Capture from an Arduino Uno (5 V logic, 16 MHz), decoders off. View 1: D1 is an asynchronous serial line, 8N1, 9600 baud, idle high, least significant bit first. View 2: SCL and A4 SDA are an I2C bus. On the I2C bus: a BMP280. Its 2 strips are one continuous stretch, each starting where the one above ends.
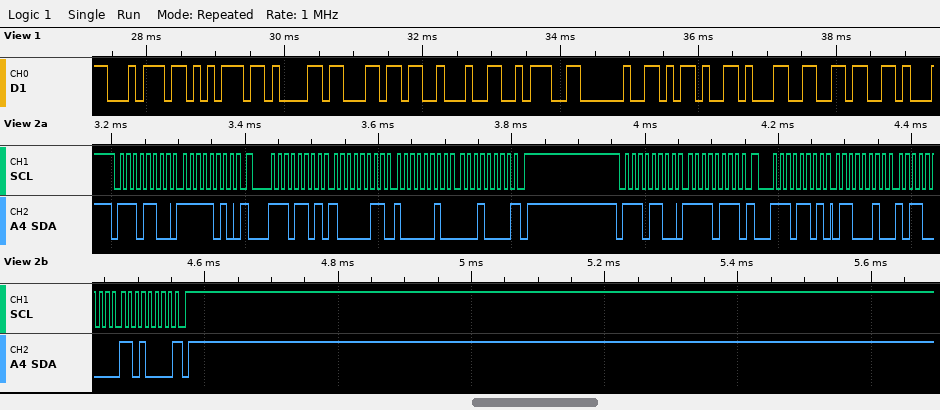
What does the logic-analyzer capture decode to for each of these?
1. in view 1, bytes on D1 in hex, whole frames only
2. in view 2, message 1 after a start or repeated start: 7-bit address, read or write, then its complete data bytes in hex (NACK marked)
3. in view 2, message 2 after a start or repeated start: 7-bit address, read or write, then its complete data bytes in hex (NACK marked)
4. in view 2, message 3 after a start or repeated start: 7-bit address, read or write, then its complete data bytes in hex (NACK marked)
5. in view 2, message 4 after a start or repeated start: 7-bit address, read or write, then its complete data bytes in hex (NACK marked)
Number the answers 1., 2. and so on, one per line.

1. 0x74 0x75 0x61 0x6C 0x22 0x3A 0x20 0x2D 0x31 0x36
2. 0x76 write: FA
3. 0x76 read: 83 82 10 NACK
4. 0x76 write: F7
5. 0x76 read: 62 B0 D0 NACK
